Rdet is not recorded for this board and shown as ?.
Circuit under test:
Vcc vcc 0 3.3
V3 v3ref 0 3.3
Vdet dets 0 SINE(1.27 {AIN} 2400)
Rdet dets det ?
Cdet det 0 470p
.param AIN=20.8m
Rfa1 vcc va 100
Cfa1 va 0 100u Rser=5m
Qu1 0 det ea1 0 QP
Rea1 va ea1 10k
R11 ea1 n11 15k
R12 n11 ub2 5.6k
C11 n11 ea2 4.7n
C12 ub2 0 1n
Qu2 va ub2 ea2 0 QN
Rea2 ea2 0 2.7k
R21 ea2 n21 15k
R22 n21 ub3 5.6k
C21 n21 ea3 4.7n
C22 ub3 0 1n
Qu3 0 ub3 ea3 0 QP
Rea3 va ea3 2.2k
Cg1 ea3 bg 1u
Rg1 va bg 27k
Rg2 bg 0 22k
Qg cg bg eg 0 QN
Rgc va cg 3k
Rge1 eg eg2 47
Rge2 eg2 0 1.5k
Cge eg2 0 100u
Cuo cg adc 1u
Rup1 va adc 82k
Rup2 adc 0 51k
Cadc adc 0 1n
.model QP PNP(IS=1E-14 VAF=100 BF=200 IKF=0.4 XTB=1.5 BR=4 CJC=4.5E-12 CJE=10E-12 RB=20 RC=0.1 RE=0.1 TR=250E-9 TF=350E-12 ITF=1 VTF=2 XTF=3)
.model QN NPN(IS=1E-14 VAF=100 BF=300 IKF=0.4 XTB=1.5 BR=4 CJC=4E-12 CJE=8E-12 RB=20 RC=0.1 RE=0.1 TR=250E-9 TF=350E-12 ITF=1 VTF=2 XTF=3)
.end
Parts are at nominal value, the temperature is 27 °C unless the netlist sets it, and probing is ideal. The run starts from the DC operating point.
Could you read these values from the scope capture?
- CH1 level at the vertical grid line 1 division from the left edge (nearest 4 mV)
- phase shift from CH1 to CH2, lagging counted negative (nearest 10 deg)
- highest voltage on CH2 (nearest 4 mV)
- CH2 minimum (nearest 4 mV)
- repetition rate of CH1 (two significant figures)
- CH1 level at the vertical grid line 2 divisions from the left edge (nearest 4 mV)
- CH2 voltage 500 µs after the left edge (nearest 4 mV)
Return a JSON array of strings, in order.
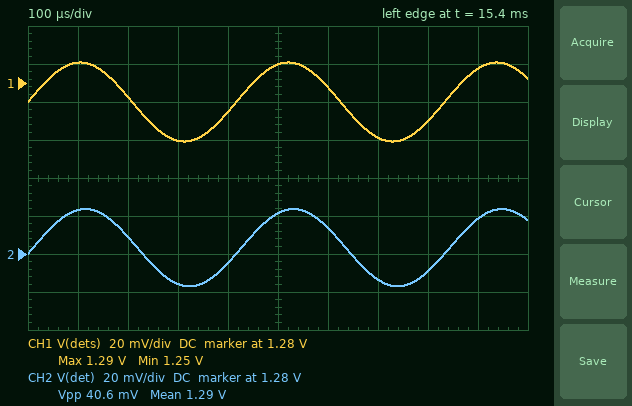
["1.292 V", "-10 deg", "1.304 V", "1.264 V", "2.4 kHz", "1.272 V", "1.300 V"]
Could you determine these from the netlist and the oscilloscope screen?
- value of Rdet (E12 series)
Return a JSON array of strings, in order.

["22 kΩ"]
